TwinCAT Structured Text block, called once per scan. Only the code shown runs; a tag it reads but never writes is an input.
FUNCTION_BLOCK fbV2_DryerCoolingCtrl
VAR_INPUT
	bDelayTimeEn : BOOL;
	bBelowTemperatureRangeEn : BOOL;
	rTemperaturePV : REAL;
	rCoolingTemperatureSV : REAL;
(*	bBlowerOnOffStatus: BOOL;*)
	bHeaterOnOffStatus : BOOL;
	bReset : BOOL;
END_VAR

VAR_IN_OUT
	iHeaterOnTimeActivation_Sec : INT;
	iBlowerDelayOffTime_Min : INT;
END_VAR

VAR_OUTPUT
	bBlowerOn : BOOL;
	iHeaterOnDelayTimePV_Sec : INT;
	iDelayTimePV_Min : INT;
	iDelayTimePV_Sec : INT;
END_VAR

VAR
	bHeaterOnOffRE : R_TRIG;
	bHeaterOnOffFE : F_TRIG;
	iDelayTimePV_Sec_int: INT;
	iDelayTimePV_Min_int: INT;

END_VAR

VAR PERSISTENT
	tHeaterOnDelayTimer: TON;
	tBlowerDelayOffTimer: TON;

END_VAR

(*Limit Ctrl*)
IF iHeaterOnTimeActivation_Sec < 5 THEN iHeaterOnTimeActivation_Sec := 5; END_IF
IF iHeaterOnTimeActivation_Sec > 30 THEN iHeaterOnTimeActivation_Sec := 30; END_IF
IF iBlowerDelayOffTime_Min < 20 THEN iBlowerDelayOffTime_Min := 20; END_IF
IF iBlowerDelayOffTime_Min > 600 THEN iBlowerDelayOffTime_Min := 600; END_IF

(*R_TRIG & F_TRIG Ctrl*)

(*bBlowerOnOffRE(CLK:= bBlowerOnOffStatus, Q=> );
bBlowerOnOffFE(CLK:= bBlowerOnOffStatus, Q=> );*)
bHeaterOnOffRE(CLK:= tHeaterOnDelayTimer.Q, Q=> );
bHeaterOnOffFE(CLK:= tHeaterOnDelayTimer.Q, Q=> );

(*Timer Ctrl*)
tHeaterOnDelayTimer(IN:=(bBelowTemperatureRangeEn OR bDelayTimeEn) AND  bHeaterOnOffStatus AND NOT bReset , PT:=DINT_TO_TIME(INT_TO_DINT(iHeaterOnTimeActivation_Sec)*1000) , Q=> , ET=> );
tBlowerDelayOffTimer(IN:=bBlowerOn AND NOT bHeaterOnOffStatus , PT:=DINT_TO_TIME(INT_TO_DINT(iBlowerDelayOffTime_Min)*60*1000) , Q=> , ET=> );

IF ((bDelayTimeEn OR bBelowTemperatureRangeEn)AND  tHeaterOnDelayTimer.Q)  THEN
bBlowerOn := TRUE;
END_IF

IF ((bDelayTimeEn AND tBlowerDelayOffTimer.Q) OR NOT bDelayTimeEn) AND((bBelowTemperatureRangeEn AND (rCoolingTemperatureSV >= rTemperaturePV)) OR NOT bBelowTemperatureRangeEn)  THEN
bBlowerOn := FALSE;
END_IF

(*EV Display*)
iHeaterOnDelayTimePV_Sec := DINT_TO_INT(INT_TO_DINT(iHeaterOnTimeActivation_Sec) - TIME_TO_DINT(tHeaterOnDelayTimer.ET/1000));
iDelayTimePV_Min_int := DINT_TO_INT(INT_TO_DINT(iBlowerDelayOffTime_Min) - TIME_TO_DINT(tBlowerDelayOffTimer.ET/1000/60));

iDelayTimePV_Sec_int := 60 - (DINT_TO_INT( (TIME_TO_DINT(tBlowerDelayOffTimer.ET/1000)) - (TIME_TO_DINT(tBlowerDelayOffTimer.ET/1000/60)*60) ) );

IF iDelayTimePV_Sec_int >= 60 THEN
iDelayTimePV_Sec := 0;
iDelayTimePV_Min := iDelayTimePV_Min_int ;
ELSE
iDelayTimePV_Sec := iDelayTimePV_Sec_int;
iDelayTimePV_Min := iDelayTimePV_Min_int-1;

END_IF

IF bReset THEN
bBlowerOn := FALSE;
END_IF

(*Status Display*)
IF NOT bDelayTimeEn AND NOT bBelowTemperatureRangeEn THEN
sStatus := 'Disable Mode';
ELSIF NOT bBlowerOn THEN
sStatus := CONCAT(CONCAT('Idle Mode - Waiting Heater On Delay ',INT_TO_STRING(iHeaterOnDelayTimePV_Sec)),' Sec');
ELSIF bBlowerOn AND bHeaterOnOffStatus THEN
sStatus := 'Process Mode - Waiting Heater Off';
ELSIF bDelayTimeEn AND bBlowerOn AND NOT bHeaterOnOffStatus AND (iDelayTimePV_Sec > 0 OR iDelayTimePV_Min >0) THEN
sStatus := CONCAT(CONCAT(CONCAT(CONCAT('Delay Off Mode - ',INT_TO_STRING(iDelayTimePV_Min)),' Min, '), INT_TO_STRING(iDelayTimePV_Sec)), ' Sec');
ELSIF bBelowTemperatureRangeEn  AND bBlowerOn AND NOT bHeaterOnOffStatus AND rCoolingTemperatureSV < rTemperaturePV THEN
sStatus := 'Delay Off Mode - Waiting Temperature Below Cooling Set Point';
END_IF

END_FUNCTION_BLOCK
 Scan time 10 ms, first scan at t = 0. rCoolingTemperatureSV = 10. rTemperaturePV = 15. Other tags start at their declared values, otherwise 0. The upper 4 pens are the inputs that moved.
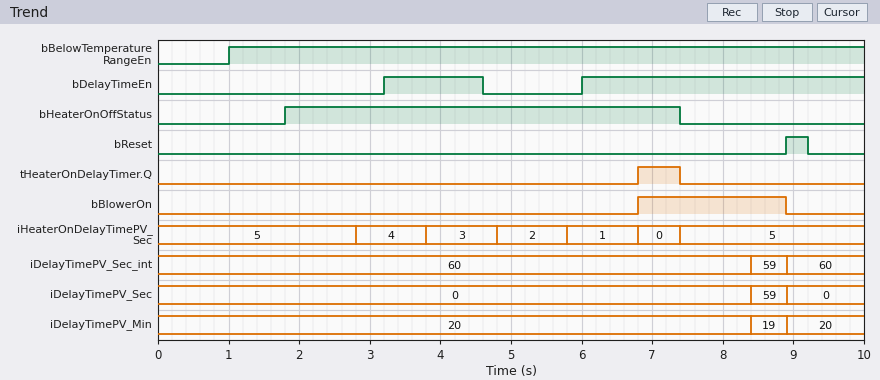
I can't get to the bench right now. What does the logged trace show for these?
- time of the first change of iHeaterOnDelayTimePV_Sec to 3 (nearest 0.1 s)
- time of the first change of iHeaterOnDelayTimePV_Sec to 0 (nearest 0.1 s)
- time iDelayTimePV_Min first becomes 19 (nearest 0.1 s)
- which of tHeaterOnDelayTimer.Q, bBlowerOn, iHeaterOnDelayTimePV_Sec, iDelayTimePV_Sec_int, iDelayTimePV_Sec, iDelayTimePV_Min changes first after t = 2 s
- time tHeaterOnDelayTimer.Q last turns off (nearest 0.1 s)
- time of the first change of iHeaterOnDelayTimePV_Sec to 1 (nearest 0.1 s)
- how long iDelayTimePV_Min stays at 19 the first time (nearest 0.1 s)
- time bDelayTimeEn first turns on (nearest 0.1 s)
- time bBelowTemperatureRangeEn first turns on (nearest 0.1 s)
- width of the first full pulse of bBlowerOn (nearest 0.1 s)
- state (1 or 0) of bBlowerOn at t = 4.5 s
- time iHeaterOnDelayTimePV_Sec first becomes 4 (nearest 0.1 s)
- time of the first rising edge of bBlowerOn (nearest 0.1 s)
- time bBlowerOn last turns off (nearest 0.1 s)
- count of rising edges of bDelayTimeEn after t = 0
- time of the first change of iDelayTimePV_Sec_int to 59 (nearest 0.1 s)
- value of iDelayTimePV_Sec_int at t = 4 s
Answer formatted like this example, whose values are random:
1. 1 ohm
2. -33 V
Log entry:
1. 3.8 s
2. 6.8 s
3. 8.4 s
4. iHeaterOnDelayTimePV_Sec
5. 7.4 s
6. 5.8 s
7. 0.5 s
8. 3.2 s
9. 1.0 s
10. 2.1 s
11. 0
12. 2.8 s
13. 6.8 s
14. 8.9 s
15. 2
16. 8.4 s
17. 60
